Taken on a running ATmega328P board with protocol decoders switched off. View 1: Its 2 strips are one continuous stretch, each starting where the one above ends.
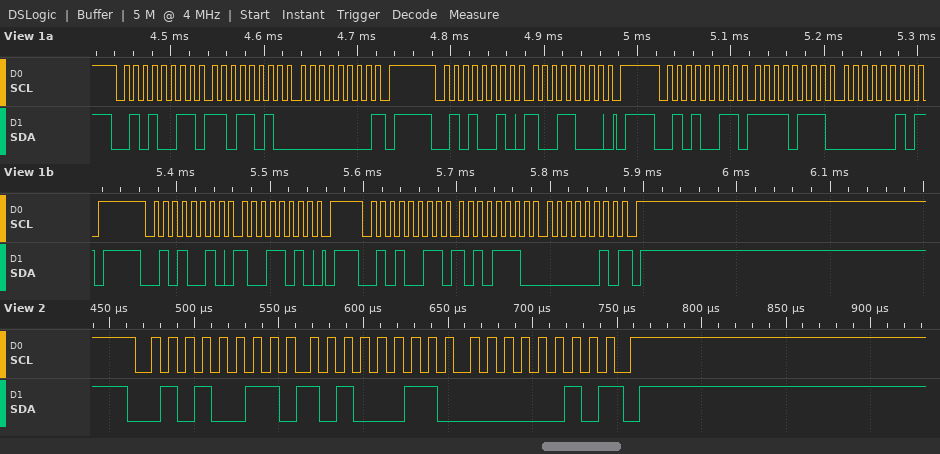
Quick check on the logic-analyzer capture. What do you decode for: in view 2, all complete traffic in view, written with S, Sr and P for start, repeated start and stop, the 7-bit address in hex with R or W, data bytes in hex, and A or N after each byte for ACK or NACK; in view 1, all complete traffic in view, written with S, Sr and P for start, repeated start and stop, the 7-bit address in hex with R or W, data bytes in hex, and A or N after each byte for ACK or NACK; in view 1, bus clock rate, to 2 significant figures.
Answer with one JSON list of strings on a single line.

["S 29R A A3 A 02 N P", "S 29R A DA A 00 N P S 29W A 98 A P S 29R A F7 A 02 N P S 29W A 9A A P S 29R A AE A 02 N P", "100 kHz"]
